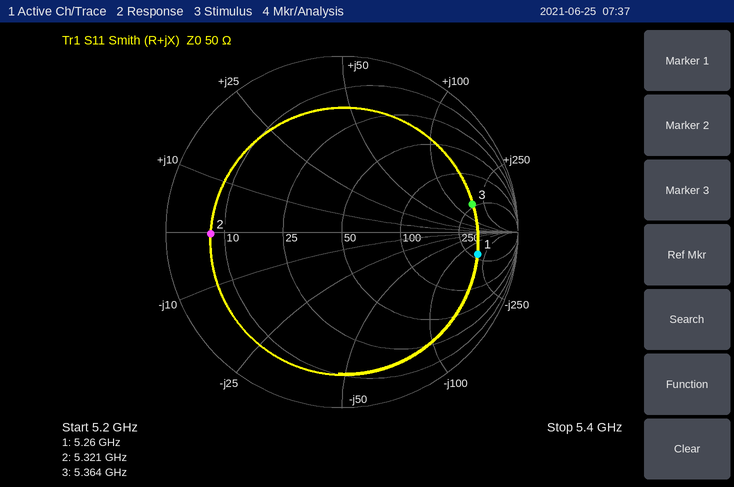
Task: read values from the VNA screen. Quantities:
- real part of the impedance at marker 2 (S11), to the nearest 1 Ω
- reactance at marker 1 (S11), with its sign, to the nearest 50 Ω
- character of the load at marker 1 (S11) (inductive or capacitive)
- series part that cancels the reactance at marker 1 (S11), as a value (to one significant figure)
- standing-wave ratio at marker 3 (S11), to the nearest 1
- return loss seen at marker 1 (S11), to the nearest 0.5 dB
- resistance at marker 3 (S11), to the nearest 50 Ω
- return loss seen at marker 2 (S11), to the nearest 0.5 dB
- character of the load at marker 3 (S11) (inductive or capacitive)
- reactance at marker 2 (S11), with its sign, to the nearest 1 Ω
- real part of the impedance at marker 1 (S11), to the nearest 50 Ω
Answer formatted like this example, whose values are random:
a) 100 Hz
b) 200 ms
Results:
a) 7 Ω
b) -200 Ω
c) capacitive
d) 6 nH
e) 7
f) 2.0 dB
g) 250 Ω
h) 2.5 dB
i) inductive
j) 0 Ω
k) 300 Ω
